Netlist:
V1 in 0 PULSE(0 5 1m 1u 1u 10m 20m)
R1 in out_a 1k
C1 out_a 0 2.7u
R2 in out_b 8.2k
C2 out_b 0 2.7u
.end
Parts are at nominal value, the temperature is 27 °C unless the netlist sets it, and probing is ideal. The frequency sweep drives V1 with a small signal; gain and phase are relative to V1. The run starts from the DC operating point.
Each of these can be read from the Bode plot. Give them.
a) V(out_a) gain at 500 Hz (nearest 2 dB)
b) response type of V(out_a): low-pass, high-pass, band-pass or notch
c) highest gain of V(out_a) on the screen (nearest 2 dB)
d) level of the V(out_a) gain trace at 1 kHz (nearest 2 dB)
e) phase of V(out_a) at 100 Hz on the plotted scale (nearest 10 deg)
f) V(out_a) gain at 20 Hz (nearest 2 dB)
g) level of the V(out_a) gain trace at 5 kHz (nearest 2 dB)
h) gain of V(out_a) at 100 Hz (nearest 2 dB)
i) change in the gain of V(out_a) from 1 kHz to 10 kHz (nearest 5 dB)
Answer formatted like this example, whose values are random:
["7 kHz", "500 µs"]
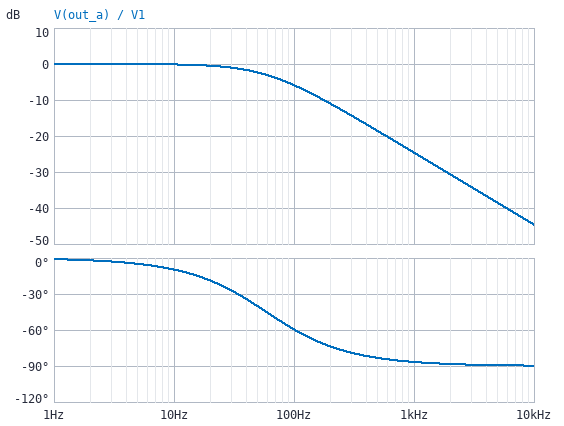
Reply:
["-18 dB", "low-pass", "0 dB", "-24 dB", "-60 deg", "0 dB", "-38 dB", "-6 dB", "-20 dB"]
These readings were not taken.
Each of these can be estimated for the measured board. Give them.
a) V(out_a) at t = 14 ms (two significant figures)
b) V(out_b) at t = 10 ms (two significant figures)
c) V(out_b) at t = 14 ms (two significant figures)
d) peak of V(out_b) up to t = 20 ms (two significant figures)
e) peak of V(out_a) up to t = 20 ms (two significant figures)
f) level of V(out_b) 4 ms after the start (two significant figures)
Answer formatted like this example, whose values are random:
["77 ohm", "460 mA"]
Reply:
["1.6 V", "1.7 V", "1.6 V", "1.8 V", "4.9 V", "630 mV"]
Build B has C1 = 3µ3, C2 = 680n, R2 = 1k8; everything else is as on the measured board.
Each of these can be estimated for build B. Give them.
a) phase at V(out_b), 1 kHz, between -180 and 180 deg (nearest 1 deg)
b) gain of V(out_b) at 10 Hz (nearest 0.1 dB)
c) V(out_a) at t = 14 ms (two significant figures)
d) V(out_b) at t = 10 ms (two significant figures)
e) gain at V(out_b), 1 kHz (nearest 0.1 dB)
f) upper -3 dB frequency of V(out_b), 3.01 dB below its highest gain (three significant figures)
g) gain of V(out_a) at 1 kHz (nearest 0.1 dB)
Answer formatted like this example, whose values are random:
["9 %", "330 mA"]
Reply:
["-83 deg", "0 dB", "1.9 V", "5.0 V", "-17.8 dB", "130 Hz", "-26.3 dB"]
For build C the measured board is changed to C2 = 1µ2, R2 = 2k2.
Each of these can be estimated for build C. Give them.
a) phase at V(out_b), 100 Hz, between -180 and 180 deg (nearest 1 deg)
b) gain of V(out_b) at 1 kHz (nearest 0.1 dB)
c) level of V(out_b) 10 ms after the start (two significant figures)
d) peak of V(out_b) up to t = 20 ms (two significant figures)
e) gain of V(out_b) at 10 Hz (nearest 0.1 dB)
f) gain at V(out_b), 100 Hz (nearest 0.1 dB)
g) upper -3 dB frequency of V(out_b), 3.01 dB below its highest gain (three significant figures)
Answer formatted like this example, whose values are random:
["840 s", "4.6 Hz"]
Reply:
["-59 deg", "-24.4 dB", "4.8 V", "4.9 V", "-0.1 dB", "-5.7 dB", "60.3 Hz"]
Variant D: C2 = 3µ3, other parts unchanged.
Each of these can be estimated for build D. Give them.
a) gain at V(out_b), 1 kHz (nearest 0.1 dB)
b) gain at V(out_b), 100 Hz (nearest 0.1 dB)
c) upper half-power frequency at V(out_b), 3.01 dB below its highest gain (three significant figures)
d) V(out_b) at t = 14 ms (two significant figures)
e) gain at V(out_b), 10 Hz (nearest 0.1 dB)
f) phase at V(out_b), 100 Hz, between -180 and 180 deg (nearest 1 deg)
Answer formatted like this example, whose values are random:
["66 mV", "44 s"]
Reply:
["-44.6 dB", "-24.6 dB", "5.88 Hz", "1.4 V", "-5.9 dB", "-87 deg"]
